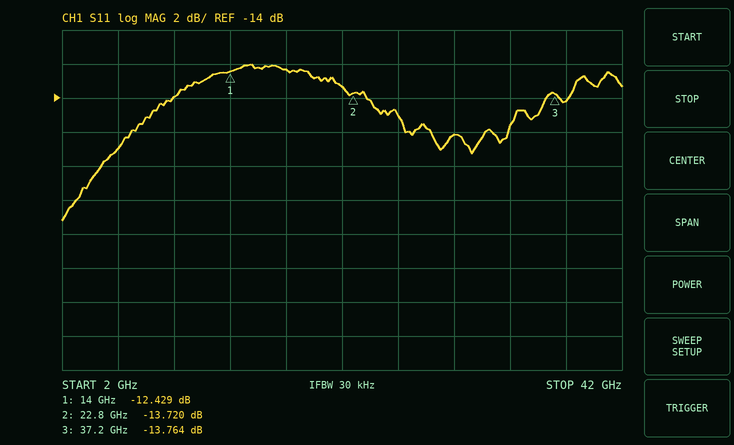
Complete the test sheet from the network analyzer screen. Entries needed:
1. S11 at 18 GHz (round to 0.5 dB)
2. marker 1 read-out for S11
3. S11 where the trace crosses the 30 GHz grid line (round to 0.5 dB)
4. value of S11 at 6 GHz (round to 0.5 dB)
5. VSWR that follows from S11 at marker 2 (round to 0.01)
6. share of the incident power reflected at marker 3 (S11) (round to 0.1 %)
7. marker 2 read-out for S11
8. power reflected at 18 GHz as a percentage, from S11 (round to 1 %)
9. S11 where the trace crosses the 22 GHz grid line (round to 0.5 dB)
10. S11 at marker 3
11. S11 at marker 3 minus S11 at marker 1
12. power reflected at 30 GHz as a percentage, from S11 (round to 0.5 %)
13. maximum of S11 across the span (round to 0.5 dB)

-12.5 dB
-12.429 dB
-16.0 dB
-17.0 dB
1.52
4.2 %
-13.720 dB
6 %
-13.5 dB
-13.764 dB
-1.335 dB
2.5 %
-12.0 dB
